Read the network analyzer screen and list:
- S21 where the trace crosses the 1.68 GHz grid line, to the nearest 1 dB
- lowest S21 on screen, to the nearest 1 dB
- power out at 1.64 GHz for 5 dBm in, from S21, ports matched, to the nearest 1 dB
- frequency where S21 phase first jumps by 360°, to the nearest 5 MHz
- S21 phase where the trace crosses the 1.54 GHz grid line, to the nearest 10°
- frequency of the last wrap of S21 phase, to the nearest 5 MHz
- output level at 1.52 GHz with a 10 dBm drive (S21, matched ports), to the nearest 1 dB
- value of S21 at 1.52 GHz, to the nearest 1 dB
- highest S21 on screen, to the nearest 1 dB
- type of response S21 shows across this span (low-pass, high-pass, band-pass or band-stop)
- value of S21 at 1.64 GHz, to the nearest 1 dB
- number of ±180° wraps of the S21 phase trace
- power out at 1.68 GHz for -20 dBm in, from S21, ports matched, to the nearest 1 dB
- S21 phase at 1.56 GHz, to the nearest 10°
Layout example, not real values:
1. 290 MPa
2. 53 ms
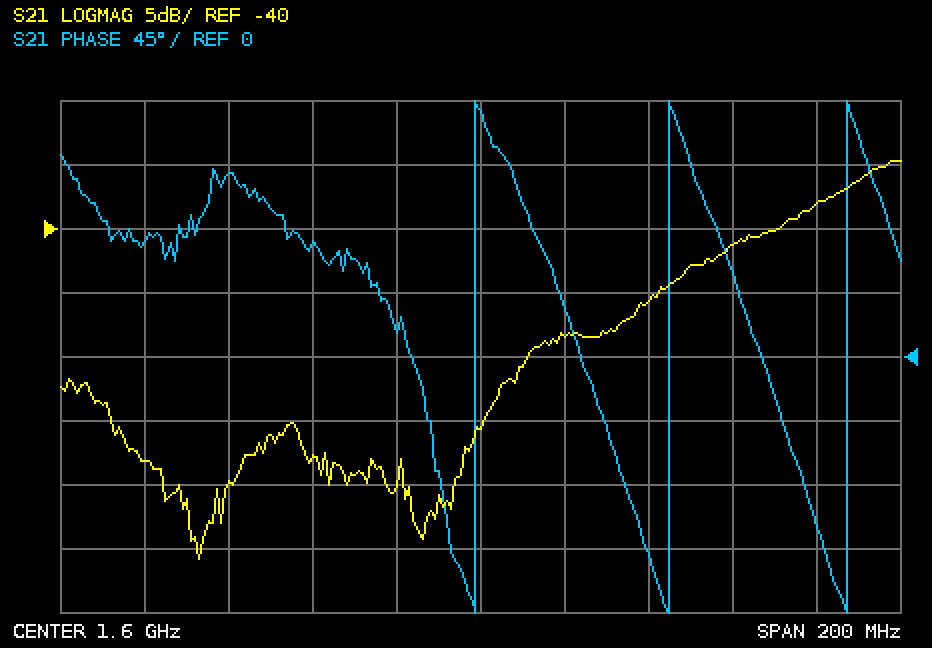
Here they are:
1. -38 dB
2. -66 dB
3. -41 dBm
4. 1.600 GHz
5. 130°
6. 1.685 GHz
7. -48 dBm
8. -58 dB
9. -35 dB
10. high-pass
11. -46 dB
12. 3
13. -58 dBm
14. 80°
